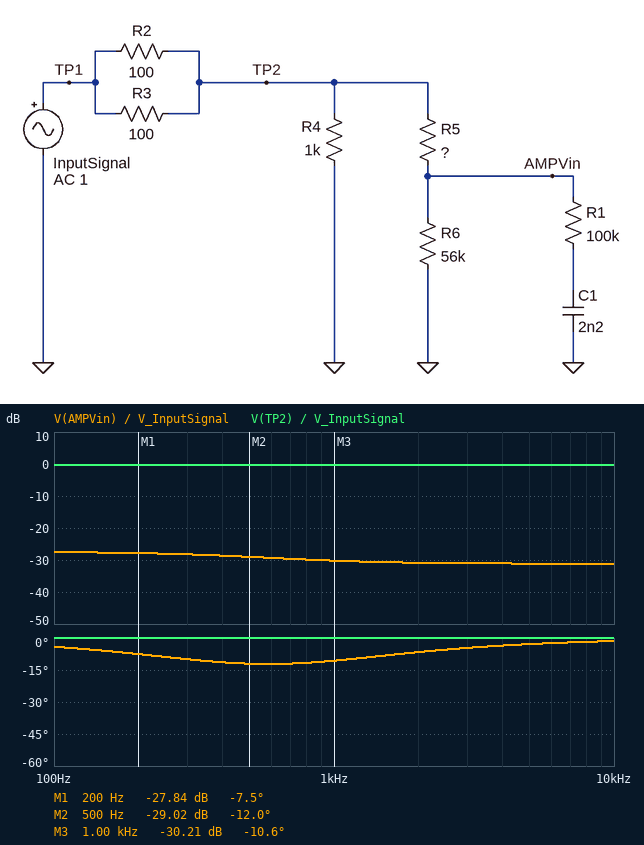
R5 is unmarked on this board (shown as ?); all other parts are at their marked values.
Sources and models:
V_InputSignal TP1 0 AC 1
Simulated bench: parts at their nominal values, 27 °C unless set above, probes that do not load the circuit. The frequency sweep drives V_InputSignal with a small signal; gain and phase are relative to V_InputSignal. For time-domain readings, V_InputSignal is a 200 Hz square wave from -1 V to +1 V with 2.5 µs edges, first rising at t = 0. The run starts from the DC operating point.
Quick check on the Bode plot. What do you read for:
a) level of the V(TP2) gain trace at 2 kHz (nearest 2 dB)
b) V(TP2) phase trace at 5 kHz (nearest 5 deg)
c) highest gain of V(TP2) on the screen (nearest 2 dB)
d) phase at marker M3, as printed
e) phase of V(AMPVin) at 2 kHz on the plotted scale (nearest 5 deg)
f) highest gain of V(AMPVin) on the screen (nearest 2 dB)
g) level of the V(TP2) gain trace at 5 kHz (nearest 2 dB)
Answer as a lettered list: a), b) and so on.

a) 0 dB
b) 0 deg
c) 0 dB
d) -10.6 deg
e) -5 deg
f) -28 dB
g) 0 dB
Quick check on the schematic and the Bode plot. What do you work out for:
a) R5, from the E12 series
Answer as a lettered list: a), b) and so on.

a) 1.2 MΩ
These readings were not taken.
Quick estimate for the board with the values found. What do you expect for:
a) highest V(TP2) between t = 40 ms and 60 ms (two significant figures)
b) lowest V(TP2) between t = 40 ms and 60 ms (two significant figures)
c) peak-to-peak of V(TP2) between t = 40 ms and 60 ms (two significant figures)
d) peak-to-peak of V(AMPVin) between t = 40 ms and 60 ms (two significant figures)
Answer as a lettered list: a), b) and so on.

a) 950 mV
b) -950 mV
c) 1.9 V
d) 85 mV
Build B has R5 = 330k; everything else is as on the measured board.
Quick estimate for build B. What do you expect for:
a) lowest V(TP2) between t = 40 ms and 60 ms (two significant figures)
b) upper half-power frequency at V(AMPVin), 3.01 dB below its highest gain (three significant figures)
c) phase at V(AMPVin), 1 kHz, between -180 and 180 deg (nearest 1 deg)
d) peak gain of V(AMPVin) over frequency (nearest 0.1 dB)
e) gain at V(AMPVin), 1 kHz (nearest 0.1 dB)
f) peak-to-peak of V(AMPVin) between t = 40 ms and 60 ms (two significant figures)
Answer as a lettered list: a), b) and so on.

a) -950 mV
b) 1.67 kHz
c) -10 deg
d) -17.2 dB
e) -19.7 dB
f) 280 mV
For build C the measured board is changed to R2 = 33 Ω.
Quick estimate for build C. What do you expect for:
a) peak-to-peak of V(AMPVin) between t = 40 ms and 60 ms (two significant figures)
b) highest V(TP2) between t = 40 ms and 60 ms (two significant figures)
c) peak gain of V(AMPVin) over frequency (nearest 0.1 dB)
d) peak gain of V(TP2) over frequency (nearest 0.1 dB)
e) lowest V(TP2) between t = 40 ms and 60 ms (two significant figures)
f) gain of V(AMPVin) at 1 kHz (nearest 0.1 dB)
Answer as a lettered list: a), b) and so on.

a) 87 mV
b) 980 mV
c) -27.2 dB
d) -0.2 dB
e) -980 mV
f) -30.0 dB
